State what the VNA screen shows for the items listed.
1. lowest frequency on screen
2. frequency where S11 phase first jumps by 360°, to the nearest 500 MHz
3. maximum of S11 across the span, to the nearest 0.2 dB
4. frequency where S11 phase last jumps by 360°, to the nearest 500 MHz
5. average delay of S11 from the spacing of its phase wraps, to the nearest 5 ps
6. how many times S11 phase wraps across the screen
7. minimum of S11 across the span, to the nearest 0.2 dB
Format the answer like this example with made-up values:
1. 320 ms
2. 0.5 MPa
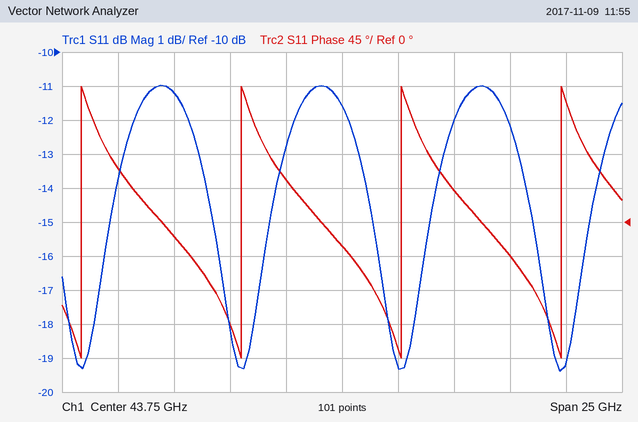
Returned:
1. 31.25 GHz
2. 32.0 GHz
3. -11.0 dB
4. 53.5 GHz
5. 140 ps
6. 4
7. -19.4 dB
